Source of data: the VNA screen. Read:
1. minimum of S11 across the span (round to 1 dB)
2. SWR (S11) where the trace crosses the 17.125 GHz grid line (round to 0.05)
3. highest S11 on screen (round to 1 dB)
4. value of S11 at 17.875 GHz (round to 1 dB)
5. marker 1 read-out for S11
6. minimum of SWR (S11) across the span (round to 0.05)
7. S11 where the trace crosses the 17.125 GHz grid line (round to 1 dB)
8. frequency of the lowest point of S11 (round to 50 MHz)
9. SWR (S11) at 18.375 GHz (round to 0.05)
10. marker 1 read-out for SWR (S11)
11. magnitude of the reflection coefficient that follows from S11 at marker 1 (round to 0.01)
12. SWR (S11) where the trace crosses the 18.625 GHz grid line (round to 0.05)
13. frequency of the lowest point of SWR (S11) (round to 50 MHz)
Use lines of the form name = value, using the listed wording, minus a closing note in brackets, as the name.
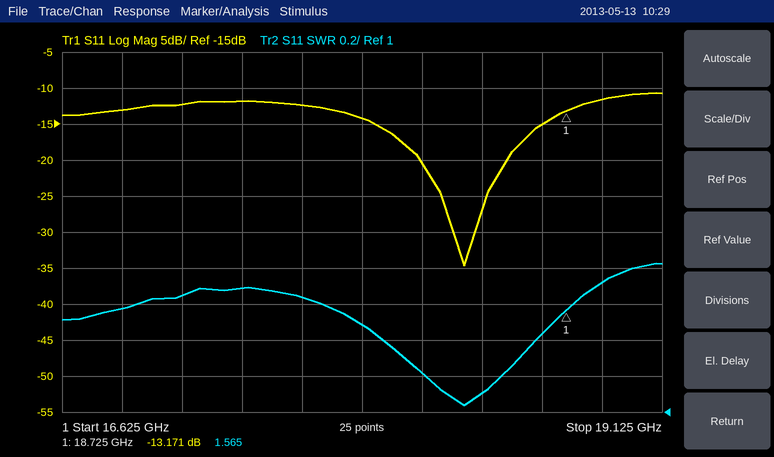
minimum of S11 across the span = -35 dB
SWR (S11) where the trace crosses the 17.125 GHz grid line = 1.65
highest S11 on screen = -11 dB
value of S11 at 17.875 GHz = -14 dB
marker 1 read-out for S11 = -13.171 dB
minimum of SWR (S11) across the span = 1.05
S11 where the trace crosses the 17.125 GHz grid line = -12 dB
frequency of the lowest point of S11 = 18.30 GHz
SWR (S11) at 18.375 GHz = 1.10
marker 1 read-out for SWR = 1.565
magnitude of the reflection coefficient that follows from S11 at marker 1 = 0.22
SWR (S11) where the trace crosses the 18.625 GHz grid line = 1.45
frequency of the lowest point of SWR (S11) = 18.30 GHz
